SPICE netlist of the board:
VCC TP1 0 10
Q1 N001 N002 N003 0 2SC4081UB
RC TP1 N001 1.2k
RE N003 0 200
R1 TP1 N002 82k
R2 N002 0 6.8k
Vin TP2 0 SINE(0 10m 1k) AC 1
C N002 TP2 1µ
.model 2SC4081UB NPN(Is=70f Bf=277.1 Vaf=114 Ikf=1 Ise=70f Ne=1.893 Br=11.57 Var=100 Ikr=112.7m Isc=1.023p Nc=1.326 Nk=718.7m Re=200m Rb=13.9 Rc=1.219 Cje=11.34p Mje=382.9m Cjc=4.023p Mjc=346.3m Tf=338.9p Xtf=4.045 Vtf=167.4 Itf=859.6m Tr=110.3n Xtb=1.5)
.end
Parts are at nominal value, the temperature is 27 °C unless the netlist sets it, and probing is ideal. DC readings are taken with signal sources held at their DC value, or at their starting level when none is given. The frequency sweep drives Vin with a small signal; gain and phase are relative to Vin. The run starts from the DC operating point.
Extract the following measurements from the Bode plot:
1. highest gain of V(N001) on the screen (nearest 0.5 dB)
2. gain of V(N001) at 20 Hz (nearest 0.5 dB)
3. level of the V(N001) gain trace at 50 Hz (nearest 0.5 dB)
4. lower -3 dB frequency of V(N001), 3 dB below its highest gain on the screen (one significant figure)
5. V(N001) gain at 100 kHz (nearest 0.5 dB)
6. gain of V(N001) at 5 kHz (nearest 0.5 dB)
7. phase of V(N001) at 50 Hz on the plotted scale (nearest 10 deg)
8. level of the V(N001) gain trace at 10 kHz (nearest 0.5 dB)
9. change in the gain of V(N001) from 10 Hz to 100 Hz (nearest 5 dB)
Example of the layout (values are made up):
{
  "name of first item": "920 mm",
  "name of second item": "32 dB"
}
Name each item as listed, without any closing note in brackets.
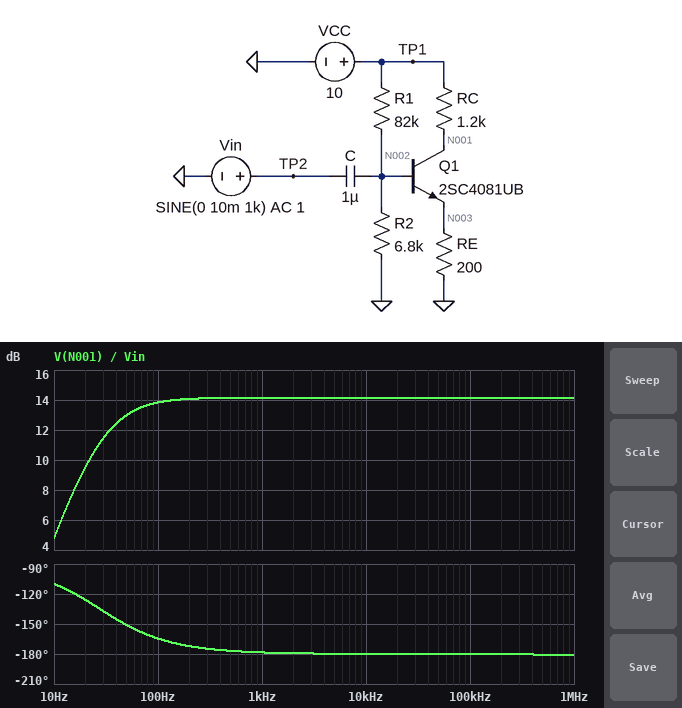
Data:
{
  "highest gain of V(N001) on the screen": "14.0 dB",
  "gain of V(N001) at 20 Hz": "9.5 dB",
  "level of the V(N001) gain trace at 50 Hz": "13.0 dB",
  "lower -3 dB frequency of V(N001), 3 dB below its highest gain on the screen": "30 Hz",
  "V(N001) gain at 100 kHz": "14.0 dB",
  "gain of V(N001) at 5 kHz": "14.0 dB",
  "phase of V(N001) at 50 Hz on the plotted scale": "-150 deg",
  "level of the V(N001) gain trace at 10 kHz": "14.0 dB",
  "change in the gain of V(N001) from 10 Hz to 100 Hz": "10 dB"
}
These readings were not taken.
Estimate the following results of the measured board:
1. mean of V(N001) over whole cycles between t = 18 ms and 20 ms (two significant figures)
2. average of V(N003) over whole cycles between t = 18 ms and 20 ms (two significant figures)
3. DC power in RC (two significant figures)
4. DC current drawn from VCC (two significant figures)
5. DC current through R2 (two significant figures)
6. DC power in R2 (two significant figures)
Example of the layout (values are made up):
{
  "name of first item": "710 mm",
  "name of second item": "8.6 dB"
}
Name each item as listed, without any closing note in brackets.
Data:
{
  "mean of V(N001) over whole cycles between t = 18 ms and 20 ms": "9.1 V",
  "average of V(N003) over whole cycles between t = 18 ms and 20 ms": "150 mV",
  "DC power in RC": "700 µW",
  "DC current drawn from VCC": "880 µA",
  "DC current through R2": "110 µA",
  "DC power in R2": "83 µW"
}
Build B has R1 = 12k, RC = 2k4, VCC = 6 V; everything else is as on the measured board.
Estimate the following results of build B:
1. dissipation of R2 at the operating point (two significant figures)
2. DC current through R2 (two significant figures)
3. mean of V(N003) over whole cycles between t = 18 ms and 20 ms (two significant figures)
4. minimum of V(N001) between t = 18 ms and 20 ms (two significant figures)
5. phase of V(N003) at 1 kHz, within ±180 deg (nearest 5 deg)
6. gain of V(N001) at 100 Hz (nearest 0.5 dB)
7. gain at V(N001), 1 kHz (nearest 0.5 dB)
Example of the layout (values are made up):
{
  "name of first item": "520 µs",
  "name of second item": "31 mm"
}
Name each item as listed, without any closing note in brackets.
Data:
{
  "dissipation of R2 at the operating point": "190 µW",
  "DC current through R2": "170 µA",
  "mean of V(N003) over whole cycles between t = 18 ms and 20 ms": "500 mV",
  "minimum of V(N001) between t = 18 ms and 20 ms": "530 mV",
  "phase of V(N003) at 1 kHz, within ±180 deg": "35 deg",
  "gain of V(N001) at 100 Hz": "-23.0 dB",
  "gain at V(N001), 1 kHz": "-8.0 dB"
}
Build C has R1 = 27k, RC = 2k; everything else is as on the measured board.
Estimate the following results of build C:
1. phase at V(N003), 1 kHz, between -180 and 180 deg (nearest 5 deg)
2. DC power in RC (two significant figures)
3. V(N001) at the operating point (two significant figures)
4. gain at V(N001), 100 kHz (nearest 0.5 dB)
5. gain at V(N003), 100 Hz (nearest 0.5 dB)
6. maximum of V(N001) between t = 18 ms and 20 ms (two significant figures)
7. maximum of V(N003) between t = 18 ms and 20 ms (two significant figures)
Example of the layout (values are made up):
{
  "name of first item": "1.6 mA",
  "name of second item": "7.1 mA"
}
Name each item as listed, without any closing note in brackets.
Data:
{
  "phase at V(N003), 1 kHz, between -180 and 180 deg": "30 deg",
  "DC power in RC": "41 mW",
  "V(N001) at the operating point": "990 mV",
  "gain at V(N001), 100 kHz": "-3.5 dB",
  "gain at V(N003), 100 Hz": "-18.0 dB",
  "maximum of V(N001) between t = 18 ms and 20 ms": "1.0 V",
  "maximum of V(N003) between t = 18 ms and 20 ms": "920 mV"
}
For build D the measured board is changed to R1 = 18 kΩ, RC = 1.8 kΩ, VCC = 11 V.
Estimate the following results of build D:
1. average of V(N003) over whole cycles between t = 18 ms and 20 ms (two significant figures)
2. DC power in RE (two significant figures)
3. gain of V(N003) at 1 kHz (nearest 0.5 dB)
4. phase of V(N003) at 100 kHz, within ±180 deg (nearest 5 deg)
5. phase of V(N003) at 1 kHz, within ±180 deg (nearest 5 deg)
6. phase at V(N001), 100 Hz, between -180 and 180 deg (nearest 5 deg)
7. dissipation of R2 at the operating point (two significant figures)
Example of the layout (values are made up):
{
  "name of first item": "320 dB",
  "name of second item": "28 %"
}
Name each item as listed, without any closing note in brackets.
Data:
{
  "average of V(N003) over whole cycles between t = 18 ms and 20 ms": "1.1 V",
  "DC power in RE": "6.5 mW",
  "gain of V(N003) at 1 kHz": "-3.5 dB",
  "phase of V(N003) at 100 kHz, within ±180 deg": "5 deg",
  "phase of V(N003) at 1 kHz, within ±180 deg": "35 deg",
  "phase at V(N001), 100 Hz, between -180 and 180 deg": "80 deg",
  "dissipation of R2 at the operating point": "480 µW"
}
